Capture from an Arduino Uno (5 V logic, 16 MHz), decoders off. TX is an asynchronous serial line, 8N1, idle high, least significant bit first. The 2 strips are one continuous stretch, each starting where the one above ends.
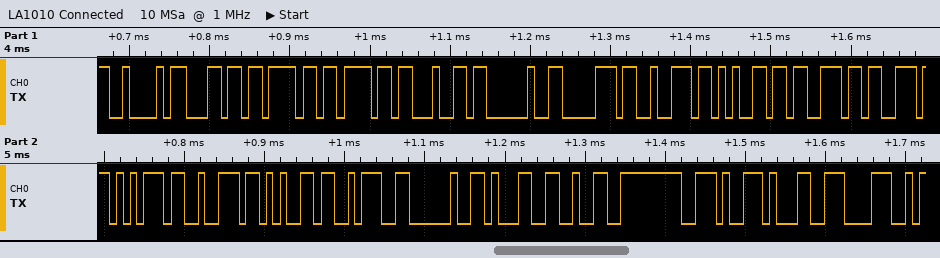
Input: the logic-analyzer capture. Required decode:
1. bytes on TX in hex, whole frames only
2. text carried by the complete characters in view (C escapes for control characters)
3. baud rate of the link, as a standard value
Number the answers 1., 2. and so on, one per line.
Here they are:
1. 42 6C 6F 6F 64 20 70 72 65 73 73 75 72 65 3A 20 31 32 2E 31 38
2. "Blood pressure: 12.18"
3. 115200 baud
